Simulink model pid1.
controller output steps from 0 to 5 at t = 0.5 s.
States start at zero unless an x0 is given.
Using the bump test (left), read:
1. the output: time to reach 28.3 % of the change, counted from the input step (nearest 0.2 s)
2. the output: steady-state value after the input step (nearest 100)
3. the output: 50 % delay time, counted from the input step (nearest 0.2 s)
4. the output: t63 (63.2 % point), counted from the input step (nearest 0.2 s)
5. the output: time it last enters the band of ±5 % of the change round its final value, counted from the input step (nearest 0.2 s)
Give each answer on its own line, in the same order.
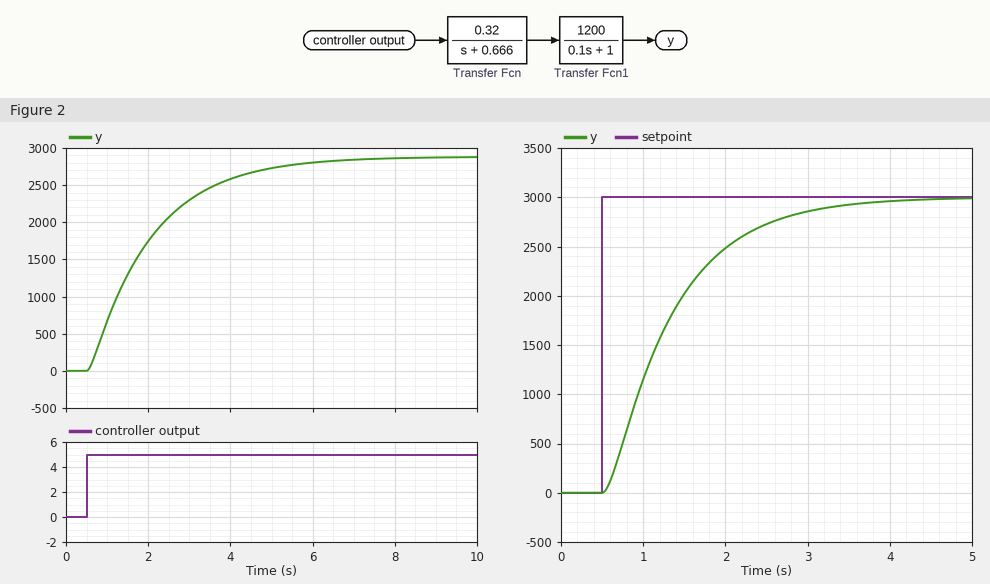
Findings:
0.6 s
2900
1.2 s
1.6 s
4.6 s
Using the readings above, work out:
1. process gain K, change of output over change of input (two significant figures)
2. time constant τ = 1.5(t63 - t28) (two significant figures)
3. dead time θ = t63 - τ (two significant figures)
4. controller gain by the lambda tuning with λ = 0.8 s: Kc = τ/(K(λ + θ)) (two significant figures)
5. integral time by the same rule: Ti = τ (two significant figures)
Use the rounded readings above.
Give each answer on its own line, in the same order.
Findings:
580
1.5 s
0.10 s
0.0029
1.5 s
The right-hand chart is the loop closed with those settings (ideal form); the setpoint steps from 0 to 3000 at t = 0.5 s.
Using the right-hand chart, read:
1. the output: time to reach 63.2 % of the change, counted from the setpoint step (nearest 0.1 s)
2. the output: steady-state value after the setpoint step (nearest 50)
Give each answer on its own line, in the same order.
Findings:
0.9 s
3000
